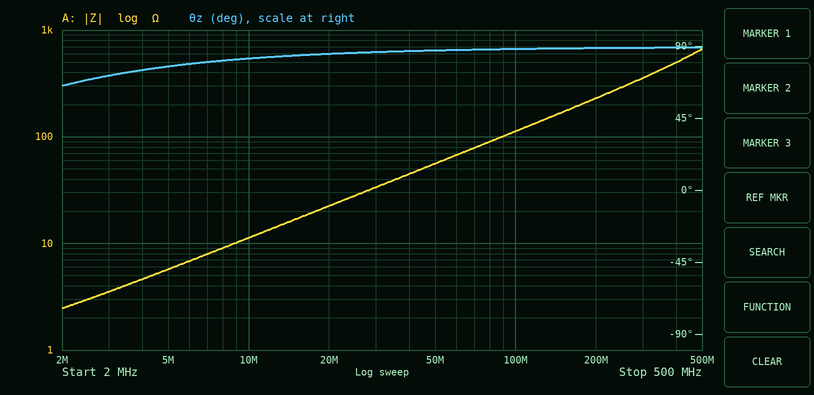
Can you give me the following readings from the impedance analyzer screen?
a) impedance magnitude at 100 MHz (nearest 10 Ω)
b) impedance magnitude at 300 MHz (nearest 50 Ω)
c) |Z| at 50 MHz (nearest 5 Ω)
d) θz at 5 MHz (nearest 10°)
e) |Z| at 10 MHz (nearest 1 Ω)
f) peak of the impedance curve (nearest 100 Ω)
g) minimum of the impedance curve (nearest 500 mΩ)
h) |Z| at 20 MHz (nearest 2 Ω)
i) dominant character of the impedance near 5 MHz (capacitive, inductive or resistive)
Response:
110 Ω
350 Ω
55 Ω
80°
11 Ω
700 Ω
2.5 Ω
22 Ω
inductive
